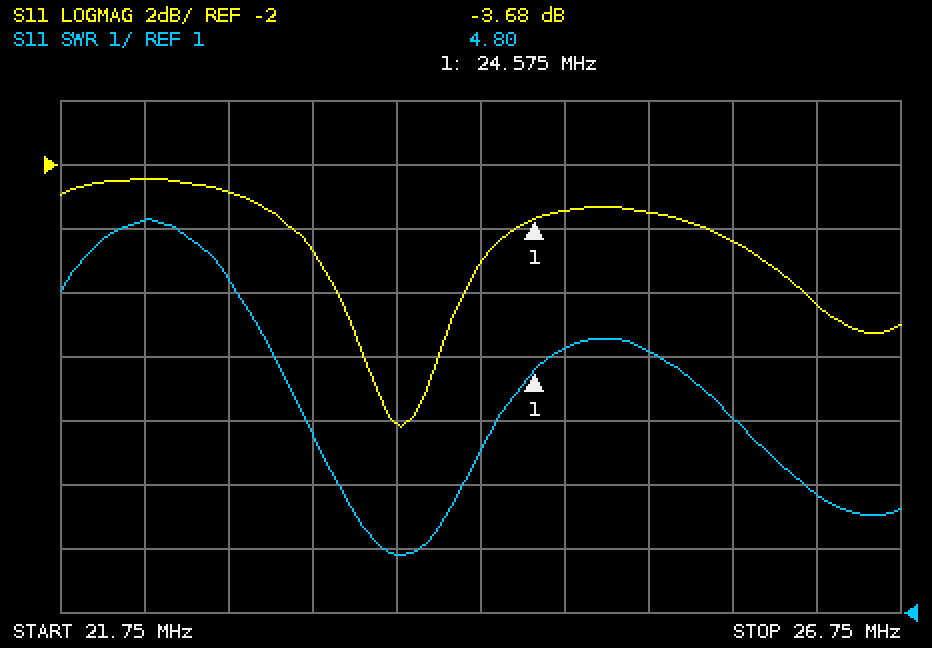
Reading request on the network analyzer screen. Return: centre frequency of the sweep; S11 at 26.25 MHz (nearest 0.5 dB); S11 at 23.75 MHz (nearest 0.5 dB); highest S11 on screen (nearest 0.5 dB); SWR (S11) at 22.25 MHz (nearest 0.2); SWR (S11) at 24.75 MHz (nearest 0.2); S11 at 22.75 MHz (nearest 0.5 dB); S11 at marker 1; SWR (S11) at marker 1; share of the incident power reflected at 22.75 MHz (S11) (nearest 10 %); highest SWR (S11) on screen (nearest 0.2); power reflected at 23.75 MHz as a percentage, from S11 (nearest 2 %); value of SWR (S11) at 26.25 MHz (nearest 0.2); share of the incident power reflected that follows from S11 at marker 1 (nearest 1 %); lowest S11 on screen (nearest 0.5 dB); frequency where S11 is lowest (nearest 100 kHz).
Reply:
24.25 MHz
-6.5 dB
-10.0 dB
-2.5 dB
7.2
5.2
-3.0 dB
-3.68 dB
4.80
50 %
7.2
10 %
2.8
43 %
-10.0 dB
23.8 MHz
